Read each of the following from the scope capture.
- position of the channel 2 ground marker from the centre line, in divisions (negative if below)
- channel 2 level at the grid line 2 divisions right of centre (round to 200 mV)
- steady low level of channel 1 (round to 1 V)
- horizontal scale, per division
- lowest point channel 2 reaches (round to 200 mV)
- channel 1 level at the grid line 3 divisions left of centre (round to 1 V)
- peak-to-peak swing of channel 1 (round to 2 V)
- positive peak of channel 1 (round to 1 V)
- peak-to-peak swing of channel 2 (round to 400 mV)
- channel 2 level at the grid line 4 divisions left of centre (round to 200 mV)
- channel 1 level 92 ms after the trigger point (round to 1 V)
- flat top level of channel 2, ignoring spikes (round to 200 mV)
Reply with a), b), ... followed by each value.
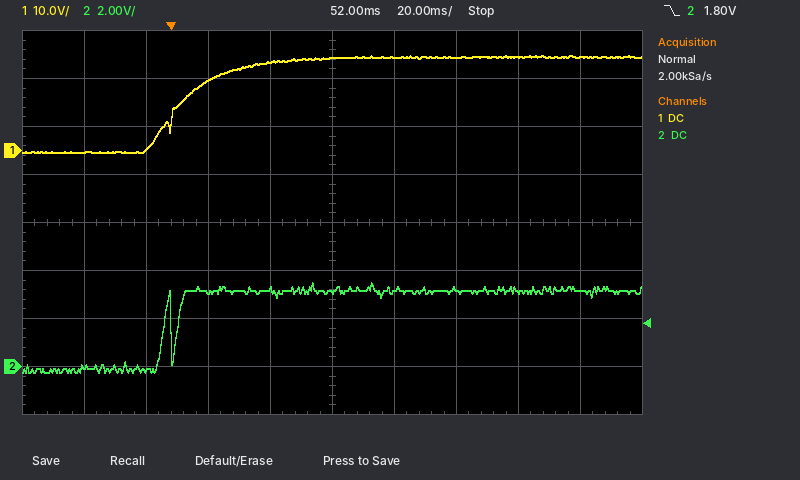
a) -3.0 div
b) 3.2 V
c) 0 V
d) 20 ms
e) -200 mV
f) 0 V
g) 20 V
h) 20 V
i) 3.6 V
j) 0.0 V
k) 19 V
l) 3.2 V
